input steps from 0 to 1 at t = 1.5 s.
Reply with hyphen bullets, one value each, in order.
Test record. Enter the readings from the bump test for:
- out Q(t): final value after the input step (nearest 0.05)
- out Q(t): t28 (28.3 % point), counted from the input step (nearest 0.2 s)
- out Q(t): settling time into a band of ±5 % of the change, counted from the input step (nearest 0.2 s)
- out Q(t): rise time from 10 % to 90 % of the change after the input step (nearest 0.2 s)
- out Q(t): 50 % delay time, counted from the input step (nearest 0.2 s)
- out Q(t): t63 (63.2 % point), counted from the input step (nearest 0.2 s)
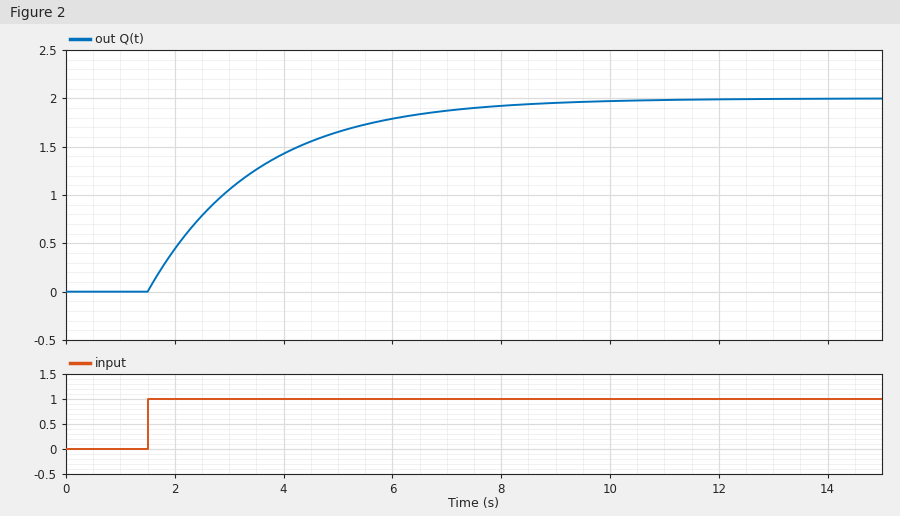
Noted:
- 2.00
- 0.6 s
- 6.0 s
- 4.4 s
- 1.4 s
- 2.0 s
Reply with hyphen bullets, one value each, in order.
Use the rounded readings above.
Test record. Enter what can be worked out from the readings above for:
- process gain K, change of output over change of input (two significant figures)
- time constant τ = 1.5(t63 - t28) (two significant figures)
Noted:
- 2.0
- 2.1 s
